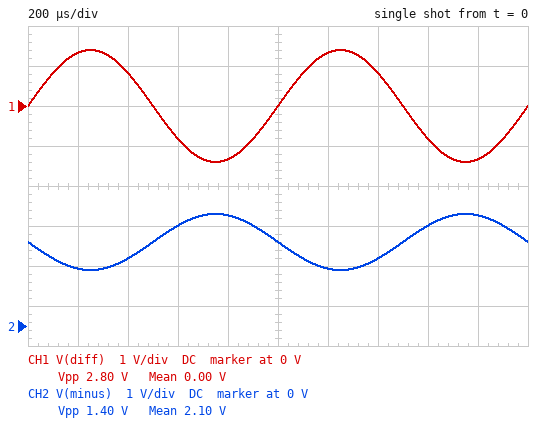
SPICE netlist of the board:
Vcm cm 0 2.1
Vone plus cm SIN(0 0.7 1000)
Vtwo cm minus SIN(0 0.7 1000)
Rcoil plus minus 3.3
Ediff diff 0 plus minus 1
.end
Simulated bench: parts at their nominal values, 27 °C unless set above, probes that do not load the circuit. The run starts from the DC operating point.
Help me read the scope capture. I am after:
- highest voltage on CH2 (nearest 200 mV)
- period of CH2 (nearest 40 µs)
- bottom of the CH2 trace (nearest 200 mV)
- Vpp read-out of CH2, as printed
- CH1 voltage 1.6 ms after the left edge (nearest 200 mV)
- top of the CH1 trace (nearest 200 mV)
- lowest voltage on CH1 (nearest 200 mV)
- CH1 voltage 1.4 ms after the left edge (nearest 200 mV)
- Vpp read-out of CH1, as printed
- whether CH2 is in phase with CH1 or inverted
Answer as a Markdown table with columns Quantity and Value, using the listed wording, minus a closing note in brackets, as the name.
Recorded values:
| Quantity | Value |
|---|---|
| highest voltage on CH2 | 2.8 V |
| period of CH2 | 1.00 ms |
| bottom of the CH2 trace | 1.4 V |
| Vpp read-out of CH2, as printed | 1.40 V |
| CH1 voltage 1.6 ms after the left edge | -800 mV |
| top of the CH1 trace | 1.4 V |
| lowest voltage on CH1 | -1.4 V |
| CH1 voltage 1.4 ms after the left edge | 800 mV |
| Vpp read-out of CH1, as printed | 2.80 V |
| whether CH2 is in phase with CH1 or inverted | inverted |
